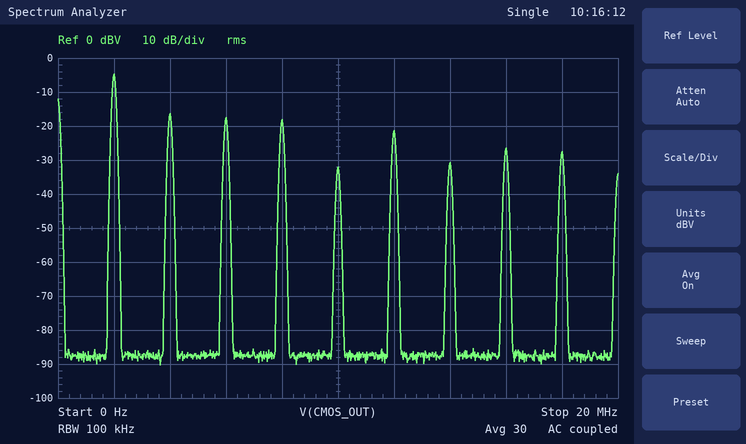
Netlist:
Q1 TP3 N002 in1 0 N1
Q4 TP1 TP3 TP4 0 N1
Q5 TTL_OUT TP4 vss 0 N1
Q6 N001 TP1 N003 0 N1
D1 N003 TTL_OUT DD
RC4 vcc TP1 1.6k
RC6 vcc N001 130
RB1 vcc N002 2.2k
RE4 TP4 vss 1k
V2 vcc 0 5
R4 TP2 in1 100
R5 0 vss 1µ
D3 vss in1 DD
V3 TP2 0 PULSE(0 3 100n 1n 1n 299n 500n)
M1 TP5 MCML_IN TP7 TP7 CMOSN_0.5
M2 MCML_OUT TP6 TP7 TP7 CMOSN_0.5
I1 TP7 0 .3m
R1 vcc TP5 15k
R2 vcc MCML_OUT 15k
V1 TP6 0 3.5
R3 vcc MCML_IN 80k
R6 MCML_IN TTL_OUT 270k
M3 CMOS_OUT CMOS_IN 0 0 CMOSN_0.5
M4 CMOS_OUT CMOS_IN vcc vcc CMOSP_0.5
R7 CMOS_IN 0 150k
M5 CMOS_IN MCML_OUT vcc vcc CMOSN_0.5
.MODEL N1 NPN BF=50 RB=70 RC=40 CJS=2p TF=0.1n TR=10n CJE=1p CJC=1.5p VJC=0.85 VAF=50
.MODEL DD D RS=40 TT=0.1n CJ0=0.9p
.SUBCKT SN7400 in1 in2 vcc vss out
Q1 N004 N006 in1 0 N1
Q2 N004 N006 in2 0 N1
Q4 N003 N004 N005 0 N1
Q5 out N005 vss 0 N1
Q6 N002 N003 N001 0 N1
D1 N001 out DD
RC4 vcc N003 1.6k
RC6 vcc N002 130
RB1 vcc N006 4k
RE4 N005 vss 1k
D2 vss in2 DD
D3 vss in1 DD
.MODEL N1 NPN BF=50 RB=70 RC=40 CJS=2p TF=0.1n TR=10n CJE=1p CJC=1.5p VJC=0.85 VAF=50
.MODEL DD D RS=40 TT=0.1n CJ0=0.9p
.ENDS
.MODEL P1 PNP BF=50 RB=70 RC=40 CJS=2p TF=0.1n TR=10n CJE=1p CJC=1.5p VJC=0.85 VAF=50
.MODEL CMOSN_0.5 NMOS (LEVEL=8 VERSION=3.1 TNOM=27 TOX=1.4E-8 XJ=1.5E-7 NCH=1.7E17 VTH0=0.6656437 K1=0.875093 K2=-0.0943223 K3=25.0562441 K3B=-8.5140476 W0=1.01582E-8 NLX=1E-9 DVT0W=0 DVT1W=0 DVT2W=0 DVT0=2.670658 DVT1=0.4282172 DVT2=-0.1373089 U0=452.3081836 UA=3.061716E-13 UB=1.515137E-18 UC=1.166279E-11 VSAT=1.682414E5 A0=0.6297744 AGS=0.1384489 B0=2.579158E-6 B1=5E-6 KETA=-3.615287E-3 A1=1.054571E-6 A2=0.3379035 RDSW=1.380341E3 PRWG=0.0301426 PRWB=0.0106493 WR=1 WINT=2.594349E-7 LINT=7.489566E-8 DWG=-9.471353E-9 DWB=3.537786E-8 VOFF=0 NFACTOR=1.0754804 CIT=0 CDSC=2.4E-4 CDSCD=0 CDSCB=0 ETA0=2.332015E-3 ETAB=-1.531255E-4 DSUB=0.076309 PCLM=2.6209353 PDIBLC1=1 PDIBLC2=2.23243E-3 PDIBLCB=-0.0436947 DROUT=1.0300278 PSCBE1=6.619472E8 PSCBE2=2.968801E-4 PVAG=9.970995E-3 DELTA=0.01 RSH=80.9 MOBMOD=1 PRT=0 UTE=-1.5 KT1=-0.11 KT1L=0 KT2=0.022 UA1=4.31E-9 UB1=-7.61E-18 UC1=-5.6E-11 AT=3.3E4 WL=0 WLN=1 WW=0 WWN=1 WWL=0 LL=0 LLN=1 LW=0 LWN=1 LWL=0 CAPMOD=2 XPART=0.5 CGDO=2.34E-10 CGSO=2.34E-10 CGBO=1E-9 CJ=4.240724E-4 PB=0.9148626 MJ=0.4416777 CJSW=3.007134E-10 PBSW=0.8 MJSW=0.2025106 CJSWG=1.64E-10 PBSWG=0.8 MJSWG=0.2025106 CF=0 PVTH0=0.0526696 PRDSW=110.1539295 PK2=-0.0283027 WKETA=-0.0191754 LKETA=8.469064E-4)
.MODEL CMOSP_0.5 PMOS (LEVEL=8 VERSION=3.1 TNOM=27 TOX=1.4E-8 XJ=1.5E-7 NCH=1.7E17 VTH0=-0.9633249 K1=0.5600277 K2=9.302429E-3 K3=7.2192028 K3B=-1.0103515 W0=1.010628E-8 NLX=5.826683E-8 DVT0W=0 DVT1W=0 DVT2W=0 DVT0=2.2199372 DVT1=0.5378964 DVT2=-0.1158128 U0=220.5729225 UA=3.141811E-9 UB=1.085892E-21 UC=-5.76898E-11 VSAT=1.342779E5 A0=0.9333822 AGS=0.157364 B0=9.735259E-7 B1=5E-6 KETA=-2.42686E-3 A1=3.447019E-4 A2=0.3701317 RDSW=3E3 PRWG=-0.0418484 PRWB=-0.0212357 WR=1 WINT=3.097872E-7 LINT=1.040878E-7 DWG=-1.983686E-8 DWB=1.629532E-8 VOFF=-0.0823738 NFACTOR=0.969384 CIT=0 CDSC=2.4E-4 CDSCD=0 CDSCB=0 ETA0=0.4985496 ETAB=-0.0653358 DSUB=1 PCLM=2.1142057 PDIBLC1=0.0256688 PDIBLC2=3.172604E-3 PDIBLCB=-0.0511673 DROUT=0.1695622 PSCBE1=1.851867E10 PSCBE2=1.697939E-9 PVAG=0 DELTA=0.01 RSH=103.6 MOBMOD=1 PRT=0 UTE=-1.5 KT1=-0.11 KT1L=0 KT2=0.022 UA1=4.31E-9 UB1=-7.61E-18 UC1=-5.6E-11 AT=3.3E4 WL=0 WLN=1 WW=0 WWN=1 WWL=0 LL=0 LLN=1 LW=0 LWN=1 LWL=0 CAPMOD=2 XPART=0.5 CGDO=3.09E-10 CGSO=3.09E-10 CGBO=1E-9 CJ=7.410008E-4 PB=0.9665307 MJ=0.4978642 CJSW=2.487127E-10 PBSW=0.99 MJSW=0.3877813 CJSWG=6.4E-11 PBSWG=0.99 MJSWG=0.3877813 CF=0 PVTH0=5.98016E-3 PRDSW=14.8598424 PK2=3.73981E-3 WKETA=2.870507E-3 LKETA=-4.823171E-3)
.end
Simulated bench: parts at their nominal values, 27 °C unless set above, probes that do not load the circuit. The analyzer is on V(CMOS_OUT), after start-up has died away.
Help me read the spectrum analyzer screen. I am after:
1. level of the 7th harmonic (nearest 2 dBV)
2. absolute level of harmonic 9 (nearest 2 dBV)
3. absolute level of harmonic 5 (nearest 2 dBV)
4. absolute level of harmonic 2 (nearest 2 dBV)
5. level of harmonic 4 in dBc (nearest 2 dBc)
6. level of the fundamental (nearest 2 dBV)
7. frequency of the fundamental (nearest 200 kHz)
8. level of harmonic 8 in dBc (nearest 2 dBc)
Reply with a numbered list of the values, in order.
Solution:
1. -30 dBV
2. -28 dBV
3. -32 dBV
4. -16 dBV
5. -14 dBc
6. -4 dBV
7. 2.0 MHz
8. -22 dBc
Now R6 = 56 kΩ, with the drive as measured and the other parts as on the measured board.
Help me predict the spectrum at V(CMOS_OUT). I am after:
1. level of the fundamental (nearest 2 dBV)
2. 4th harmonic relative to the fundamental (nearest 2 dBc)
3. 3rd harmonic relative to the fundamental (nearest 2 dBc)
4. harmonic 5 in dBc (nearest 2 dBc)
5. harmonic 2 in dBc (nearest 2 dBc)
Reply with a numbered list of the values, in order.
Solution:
1. 6 dBV
2. -12 dBc
3. -20 dBc
4. -18 dBc
5. -8 dBc
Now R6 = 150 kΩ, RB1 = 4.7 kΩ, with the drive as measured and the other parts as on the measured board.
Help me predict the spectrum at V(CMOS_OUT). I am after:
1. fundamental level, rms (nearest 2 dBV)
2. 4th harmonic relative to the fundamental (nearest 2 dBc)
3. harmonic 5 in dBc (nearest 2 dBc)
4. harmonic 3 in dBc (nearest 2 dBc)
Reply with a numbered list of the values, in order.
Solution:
1. 6 dBV
2. -12 dBc
3. -24 dBc
4. -16 dBc
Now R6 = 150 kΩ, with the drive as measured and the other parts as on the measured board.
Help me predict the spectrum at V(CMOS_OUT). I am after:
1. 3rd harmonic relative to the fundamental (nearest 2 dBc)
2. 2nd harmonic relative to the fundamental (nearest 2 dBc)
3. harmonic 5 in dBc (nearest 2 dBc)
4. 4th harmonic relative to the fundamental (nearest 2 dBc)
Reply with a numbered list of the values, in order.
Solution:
1. -18 dBc
2. -8 dBc
3. -22 dBc
4. -12 dBc
